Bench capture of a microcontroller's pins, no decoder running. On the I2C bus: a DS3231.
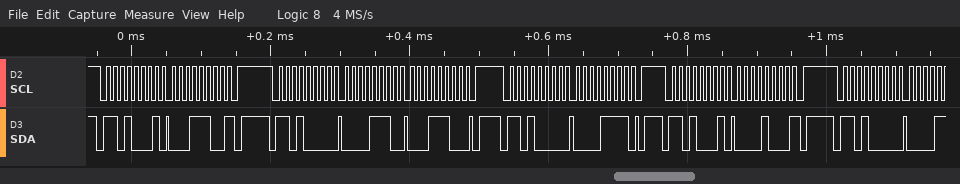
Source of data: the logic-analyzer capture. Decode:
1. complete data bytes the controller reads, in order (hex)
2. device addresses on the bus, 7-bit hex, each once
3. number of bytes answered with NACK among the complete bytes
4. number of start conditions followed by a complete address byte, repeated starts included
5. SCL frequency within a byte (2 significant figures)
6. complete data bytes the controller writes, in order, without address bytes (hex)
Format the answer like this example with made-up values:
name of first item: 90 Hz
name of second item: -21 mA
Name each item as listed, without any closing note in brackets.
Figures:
complete data bytes the controller reads, in order: 1C 08
device addresses on the bus, 7-bit hex, each once: 0x68
number of bytes answered with NACK among the complete bytes: 2
number of start conditions followed by a complete address byte, repeated starts included: 5
SCL frequency within a byte: 100 kHz
complete data bytes the controller writes, in order, without address bytes: 0E 1C 0F
